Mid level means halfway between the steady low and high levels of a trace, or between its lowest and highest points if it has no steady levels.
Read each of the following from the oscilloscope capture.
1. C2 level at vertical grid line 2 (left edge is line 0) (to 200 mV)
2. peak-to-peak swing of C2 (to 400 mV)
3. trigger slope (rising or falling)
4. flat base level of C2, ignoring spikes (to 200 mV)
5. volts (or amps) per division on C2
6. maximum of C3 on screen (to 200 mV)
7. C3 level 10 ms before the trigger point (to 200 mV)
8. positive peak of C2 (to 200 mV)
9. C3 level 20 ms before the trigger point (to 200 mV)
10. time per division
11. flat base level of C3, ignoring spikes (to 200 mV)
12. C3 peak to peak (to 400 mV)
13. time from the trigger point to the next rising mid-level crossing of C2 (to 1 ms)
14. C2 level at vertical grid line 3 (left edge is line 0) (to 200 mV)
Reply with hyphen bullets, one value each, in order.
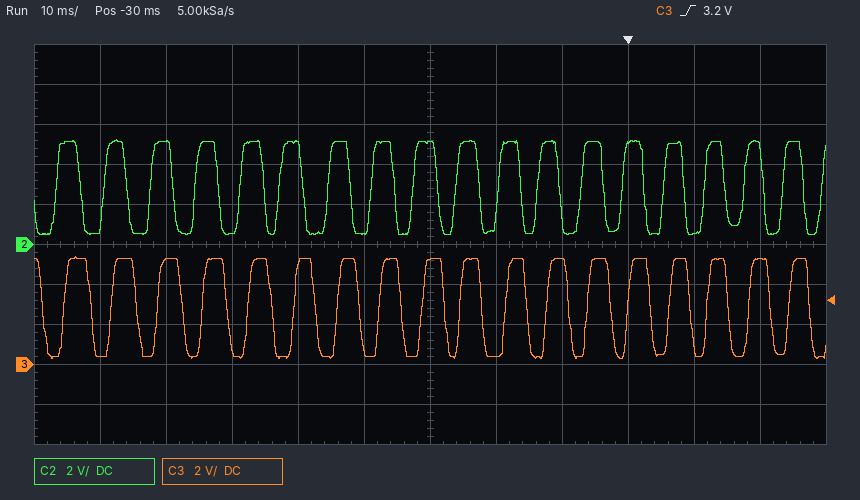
- 5.2 V
- 4.8 V
- rising
- 600 mV
- 2 V
- 5.4 V
- 5.2 V
- 5.2 V
- 400 mV
- 10 ms
- 400 mV
- 5.2 V
- 5 ms
- 600 mV
